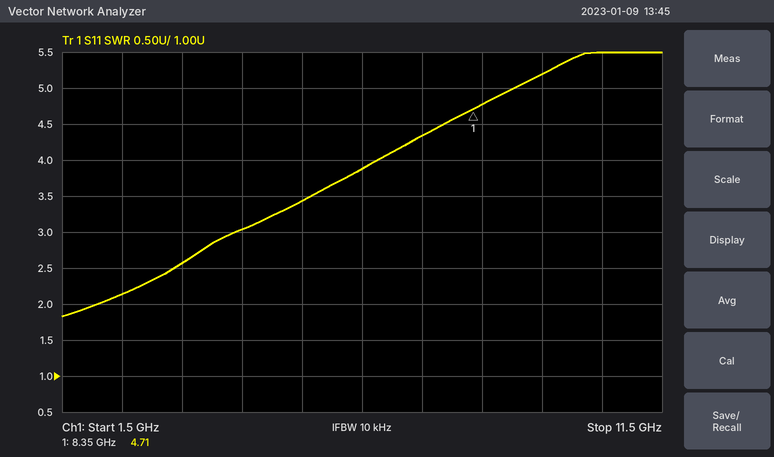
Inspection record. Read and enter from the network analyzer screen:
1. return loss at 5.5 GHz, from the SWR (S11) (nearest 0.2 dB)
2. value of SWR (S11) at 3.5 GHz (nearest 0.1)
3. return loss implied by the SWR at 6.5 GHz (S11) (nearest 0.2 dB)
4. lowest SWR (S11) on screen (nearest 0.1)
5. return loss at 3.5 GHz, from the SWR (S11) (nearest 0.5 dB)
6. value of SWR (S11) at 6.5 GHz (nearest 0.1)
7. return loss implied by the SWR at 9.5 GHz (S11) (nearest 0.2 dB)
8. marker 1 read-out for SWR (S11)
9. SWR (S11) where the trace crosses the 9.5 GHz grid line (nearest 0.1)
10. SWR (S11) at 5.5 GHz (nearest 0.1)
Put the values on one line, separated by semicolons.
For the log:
5.2 dB; 2.6; 4.6 dB; 1.8; 7.0 dB; 3.9; 3.4 dB; 4.71; 5.2; 3.4
